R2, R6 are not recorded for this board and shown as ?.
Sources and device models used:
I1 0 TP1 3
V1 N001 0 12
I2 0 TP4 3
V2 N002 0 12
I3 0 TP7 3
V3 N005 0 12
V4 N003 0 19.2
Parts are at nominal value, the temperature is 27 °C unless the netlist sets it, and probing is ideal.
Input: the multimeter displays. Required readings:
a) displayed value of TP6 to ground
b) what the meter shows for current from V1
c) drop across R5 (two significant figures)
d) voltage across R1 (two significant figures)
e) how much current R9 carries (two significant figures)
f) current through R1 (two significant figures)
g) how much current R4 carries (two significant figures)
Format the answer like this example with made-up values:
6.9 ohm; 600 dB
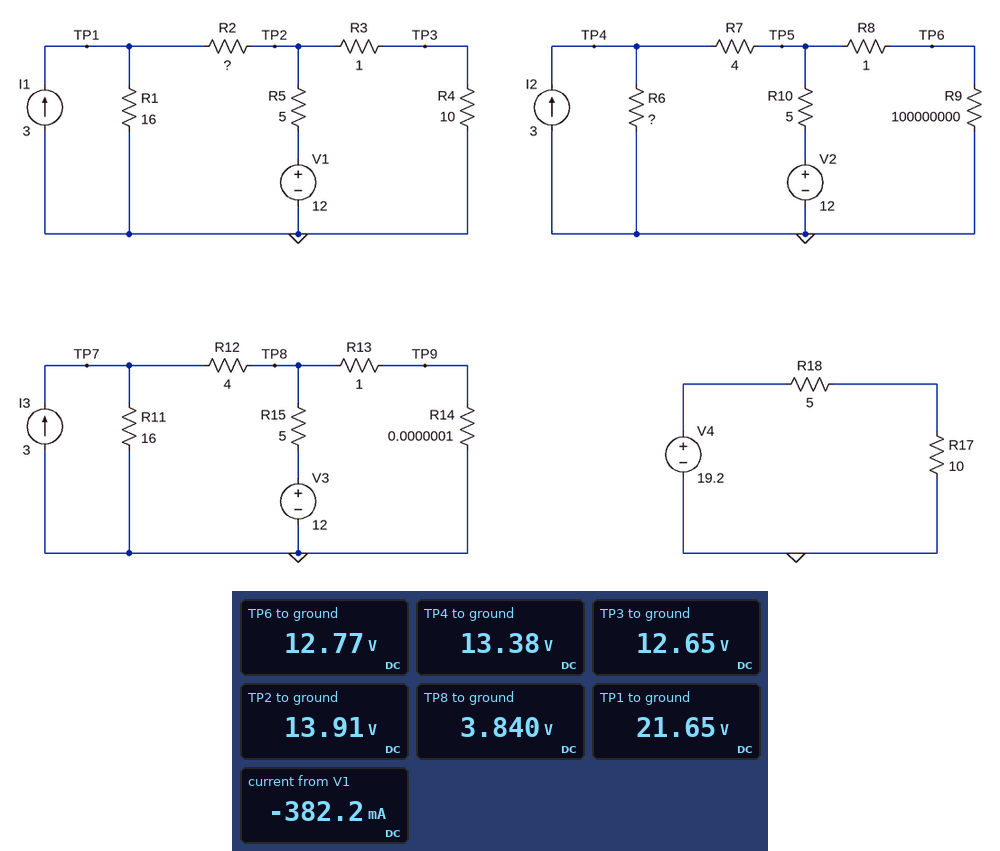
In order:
12.77 V; -382.2 mA; 1.9 V; 22 V; 130 nA; 1.4 A; 1.3 A
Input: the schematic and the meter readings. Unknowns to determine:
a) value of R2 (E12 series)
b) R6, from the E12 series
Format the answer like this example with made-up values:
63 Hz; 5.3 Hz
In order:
4.7 Ω; 4.7 Ω
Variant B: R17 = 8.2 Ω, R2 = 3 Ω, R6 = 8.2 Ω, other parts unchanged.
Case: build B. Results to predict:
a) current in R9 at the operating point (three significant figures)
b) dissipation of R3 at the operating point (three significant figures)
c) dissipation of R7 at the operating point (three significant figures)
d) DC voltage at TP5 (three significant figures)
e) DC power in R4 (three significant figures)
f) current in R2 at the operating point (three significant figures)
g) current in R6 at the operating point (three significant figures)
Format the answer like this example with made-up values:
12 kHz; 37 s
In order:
157 nA; 1.70 W; 2.15 W; 15.7 V; 17.0 W; 1.77 A; 2.27 A
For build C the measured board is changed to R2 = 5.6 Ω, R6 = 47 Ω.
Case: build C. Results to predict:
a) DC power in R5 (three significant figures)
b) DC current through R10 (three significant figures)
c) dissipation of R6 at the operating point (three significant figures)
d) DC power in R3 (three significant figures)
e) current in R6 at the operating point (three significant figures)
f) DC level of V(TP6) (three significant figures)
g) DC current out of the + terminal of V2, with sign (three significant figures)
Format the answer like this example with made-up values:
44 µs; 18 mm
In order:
583 mW; 2.30 A; 22.8 W; 1.55 W; 696 mA; 23.5 V; -2.30 A
